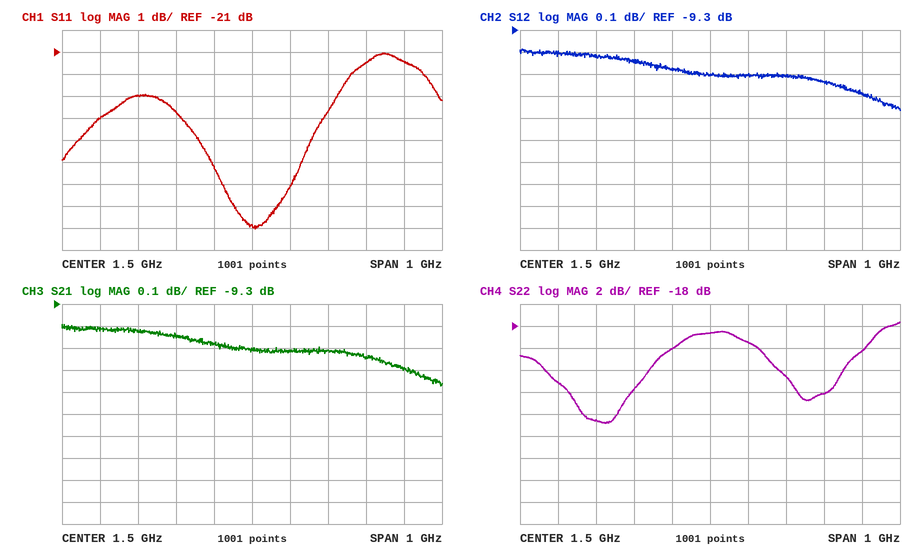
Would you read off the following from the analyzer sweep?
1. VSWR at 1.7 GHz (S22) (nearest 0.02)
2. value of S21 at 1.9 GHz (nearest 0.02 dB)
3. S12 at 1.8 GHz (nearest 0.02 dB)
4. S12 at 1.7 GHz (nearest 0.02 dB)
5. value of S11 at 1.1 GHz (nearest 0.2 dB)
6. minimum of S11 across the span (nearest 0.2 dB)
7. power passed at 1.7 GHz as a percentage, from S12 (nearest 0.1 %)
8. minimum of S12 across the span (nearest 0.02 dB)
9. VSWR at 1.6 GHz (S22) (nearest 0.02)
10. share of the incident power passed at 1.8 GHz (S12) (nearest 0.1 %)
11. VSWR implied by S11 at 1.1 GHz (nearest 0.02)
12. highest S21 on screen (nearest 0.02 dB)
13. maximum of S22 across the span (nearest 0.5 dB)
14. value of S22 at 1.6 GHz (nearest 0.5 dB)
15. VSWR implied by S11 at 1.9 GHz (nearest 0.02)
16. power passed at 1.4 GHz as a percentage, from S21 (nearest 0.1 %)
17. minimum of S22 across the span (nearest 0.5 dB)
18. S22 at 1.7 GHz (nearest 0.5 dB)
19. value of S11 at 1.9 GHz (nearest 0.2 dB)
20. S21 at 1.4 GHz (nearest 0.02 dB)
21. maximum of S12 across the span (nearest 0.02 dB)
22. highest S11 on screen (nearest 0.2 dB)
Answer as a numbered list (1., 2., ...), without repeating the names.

1. 1.16
2. -9.60 dB
3. -9.54 dB
4. -9.50 dB
5. -24.0 dB
6. -29.0 dB
7. 11.2 %
8. -9.66 dB
9. 1.24
10. 11.1 %
11. 1.14
12. -9.40 dB
13. -17.5 dB
14. -19.5 dB
15. 1.18
16. 11.3 %
17. -27.0 dB
18. -22.5 dB
19. -21.4 dB
20. -9.48 dB
21. -9.38 dB
22. -21.0 dB
